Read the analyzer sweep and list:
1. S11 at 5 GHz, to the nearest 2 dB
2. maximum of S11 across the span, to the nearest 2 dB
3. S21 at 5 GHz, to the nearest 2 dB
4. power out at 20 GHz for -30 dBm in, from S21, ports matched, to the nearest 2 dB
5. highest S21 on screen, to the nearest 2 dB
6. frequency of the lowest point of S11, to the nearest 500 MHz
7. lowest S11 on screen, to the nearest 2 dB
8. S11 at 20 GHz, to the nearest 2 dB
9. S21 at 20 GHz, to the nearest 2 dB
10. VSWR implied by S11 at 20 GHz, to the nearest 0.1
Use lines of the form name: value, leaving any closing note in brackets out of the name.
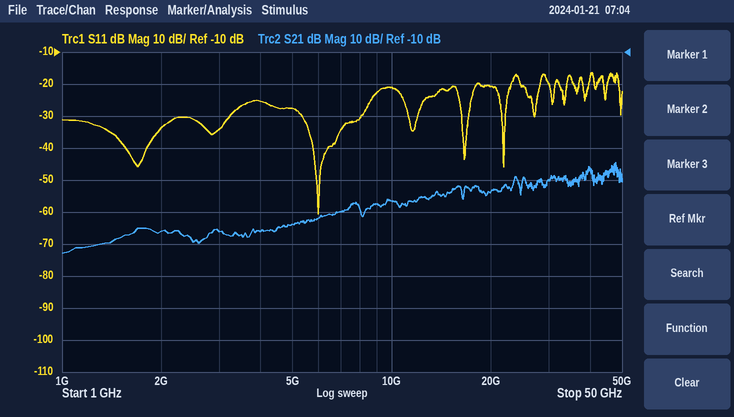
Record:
S11 at 5 GHz, to the nearest 2 dB: -28 dB
maximum of S11 across the span, to the nearest 2 dB: -16 dB
S21 at 5 GHz, to the nearest 2 dB: -64 dB
power out at 20 GHz for -30 dBm in, from S21, ports matched, to the nearest 2 dB: -84 dBm
highest S21 on screen, to the nearest 2 dB: -44 dB
frequency of the lowest point of S11, to the nearest 500 MHz: 6.0 GHz
lowest S11 on screen, to the nearest 2 dB: -60 dB
S11 at 20 GHz, to the nearest 2 dB: -20 dB
S21 at 20 GHz, to the nearest 2 dB: -54 dB
VSWR implied by S11 at 20 GHz, to the nearest 0.1: 1.2
